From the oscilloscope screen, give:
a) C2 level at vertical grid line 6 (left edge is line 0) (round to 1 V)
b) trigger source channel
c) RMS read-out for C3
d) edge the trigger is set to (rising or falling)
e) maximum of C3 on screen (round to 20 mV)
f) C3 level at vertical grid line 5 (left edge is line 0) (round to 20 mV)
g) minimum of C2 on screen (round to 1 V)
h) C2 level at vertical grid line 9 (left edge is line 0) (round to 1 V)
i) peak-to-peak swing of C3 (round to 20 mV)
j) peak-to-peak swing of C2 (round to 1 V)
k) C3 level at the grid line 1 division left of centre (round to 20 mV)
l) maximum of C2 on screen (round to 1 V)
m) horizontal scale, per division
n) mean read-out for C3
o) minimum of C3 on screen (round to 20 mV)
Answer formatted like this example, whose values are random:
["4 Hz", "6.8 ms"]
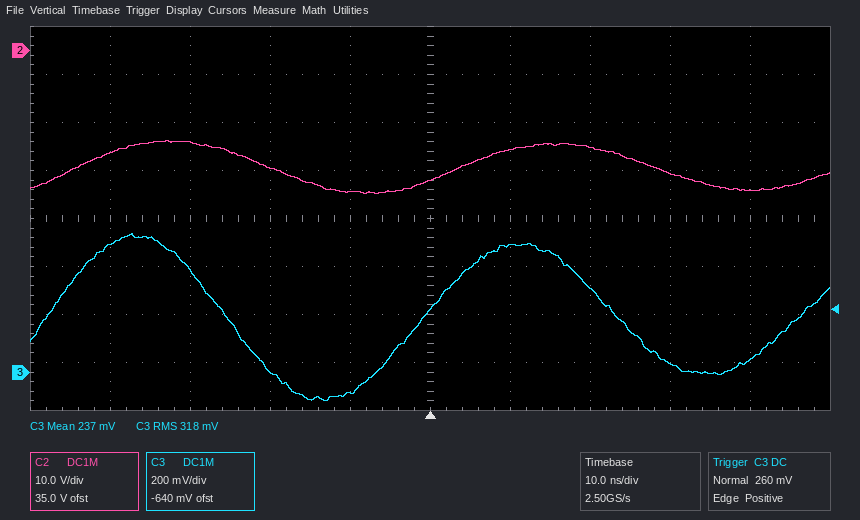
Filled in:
["-21 V", "C3", "318 mV", "rising", "580 mV", "260 mV", "-30 V", "-29 V", "700 mV", "11 V", "-80 mV", "-19 V", "10 ns", "237 mV", "-120 mV"]
